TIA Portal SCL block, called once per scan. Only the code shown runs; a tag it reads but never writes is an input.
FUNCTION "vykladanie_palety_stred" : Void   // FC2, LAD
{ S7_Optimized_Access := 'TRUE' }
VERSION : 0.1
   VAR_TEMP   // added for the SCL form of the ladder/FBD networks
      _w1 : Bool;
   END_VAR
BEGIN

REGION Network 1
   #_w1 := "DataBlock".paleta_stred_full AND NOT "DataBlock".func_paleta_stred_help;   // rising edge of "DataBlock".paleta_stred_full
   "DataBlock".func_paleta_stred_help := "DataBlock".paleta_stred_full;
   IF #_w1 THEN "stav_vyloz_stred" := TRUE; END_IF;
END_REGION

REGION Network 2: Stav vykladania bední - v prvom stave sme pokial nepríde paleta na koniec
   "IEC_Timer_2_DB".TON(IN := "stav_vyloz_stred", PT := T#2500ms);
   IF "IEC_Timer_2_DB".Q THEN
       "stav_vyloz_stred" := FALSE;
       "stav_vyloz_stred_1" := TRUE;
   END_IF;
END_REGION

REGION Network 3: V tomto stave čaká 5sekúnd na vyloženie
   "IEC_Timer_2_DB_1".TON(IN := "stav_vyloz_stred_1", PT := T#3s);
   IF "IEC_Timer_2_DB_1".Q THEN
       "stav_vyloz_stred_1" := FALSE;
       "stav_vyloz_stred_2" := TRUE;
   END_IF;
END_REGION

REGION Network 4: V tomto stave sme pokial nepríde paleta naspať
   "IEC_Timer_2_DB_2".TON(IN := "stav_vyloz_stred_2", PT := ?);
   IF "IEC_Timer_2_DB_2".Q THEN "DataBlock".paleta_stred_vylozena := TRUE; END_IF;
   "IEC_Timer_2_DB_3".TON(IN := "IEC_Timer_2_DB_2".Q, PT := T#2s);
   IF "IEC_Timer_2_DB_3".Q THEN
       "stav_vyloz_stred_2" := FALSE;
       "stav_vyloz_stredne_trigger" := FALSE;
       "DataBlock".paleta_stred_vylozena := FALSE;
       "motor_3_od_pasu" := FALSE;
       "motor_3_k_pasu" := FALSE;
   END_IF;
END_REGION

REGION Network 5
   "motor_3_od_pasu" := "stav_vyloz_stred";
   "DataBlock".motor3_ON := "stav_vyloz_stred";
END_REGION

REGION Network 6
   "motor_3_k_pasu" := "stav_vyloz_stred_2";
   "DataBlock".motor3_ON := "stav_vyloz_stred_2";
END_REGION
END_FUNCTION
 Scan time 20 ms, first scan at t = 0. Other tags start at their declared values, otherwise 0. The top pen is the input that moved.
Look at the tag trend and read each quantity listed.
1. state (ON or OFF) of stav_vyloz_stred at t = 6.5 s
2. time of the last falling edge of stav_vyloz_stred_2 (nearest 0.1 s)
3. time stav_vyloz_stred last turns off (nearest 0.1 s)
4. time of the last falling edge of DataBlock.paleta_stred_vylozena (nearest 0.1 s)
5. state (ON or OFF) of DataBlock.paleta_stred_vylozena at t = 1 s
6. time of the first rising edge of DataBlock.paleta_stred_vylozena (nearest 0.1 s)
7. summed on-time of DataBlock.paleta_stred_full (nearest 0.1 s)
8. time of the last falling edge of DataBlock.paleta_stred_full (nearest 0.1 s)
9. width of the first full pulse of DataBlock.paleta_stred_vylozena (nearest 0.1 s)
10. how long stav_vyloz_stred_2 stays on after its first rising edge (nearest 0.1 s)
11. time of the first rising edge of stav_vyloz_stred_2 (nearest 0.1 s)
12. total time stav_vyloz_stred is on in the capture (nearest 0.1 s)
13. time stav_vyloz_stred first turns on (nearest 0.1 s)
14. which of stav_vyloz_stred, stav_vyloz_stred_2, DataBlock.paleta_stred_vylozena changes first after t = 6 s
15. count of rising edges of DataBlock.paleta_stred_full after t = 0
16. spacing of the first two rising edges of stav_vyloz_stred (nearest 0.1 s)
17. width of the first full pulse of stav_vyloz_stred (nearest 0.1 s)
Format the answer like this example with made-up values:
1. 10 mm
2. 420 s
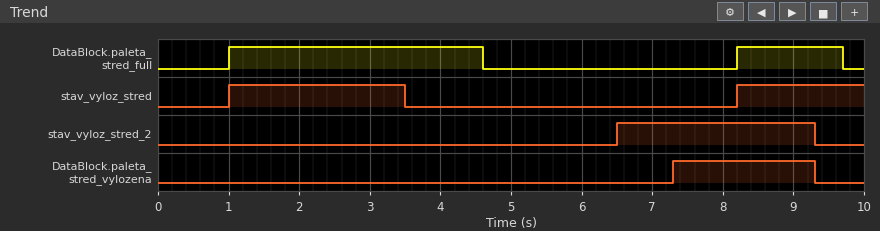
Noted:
1. OFF
2. 9.3 s
3. 3.5 s
4. 9.3 s
5. OFF
6. 7.3 s
7. 5.1 s
8. 9.7 s
9. 2.0 s
10. 2.8 s
11. 6.5 s
12. 4.3 s
13. 1.0 s
14. stav_vyloz_stred_2
15. 2
16. 7.2 s
17. 2.5 s
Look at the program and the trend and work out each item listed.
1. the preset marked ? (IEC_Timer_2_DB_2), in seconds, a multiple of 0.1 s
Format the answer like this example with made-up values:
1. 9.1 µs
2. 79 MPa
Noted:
1. 0.8 s
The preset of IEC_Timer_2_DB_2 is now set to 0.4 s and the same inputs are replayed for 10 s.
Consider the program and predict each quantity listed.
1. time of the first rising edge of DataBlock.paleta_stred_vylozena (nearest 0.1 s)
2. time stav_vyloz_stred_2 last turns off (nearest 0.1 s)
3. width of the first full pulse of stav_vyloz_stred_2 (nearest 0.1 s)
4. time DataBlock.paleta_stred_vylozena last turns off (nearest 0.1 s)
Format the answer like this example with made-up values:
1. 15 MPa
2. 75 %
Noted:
1. 6.9 s
2. 8.9 s
3. 2.4 s
4. 8.9 s
